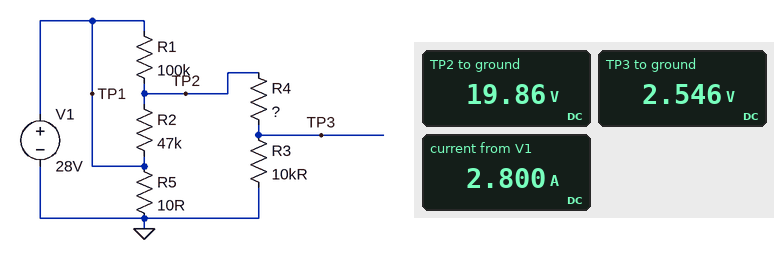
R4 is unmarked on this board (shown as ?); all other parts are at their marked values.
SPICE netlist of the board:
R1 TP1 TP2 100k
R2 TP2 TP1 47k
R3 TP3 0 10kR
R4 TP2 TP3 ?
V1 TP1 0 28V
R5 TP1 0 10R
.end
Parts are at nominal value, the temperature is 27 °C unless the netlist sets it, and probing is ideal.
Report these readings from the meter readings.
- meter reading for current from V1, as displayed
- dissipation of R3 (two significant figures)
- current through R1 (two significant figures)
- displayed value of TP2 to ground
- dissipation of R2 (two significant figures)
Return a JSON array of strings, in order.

["2.800 A", "650 µW", "81 µA", "19.86 V", "1.4 mW"]
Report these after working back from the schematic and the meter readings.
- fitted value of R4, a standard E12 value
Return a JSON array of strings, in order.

["68 kΩ"]
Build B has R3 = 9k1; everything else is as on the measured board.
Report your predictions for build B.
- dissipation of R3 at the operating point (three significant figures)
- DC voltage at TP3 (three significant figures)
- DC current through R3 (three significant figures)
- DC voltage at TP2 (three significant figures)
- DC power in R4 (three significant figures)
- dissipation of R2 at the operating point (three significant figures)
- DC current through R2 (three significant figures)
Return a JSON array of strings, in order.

["600 µW", "2.34 V", "257 µA", "19.8 V", "4.48 mW", "1.43 mW", "175 µA"]
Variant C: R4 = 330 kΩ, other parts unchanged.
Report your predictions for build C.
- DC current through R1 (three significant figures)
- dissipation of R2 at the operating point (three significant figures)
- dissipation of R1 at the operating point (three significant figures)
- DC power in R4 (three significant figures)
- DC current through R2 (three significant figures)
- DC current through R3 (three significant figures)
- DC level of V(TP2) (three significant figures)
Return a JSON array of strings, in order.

["24.1 µA", "123 µW", "57.9 µW", "1.87 mW", "51.2 µA", "75.3 µA", "25.6 V"]
